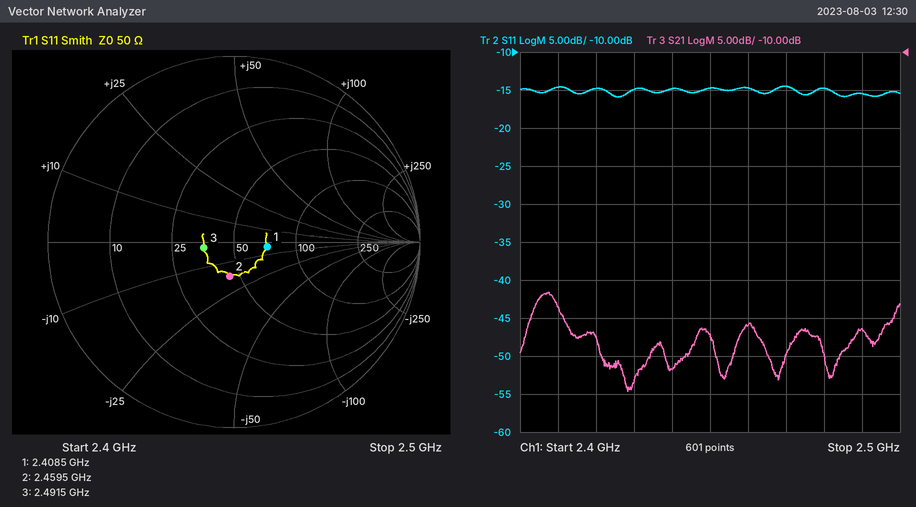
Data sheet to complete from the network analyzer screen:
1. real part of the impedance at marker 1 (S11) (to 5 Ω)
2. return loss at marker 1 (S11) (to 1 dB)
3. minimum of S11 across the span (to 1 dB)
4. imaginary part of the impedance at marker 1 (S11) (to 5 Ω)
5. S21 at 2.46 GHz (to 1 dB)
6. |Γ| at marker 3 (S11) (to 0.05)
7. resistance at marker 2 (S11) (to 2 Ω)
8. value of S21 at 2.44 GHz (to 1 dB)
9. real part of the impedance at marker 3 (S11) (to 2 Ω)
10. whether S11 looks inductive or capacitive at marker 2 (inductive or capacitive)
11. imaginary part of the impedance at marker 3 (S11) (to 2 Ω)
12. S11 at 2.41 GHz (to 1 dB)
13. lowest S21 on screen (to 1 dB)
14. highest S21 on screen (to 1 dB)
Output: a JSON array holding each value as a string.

["70 Ω", "15 dB", "-16 dB", "-5 Ω", "-46 dB", "0.15", "44 Ω", "-52 dB", "36 Ω", "capacitive", "-2 Ω", "-15 dB", "-55 dB", "-42 dB"]
